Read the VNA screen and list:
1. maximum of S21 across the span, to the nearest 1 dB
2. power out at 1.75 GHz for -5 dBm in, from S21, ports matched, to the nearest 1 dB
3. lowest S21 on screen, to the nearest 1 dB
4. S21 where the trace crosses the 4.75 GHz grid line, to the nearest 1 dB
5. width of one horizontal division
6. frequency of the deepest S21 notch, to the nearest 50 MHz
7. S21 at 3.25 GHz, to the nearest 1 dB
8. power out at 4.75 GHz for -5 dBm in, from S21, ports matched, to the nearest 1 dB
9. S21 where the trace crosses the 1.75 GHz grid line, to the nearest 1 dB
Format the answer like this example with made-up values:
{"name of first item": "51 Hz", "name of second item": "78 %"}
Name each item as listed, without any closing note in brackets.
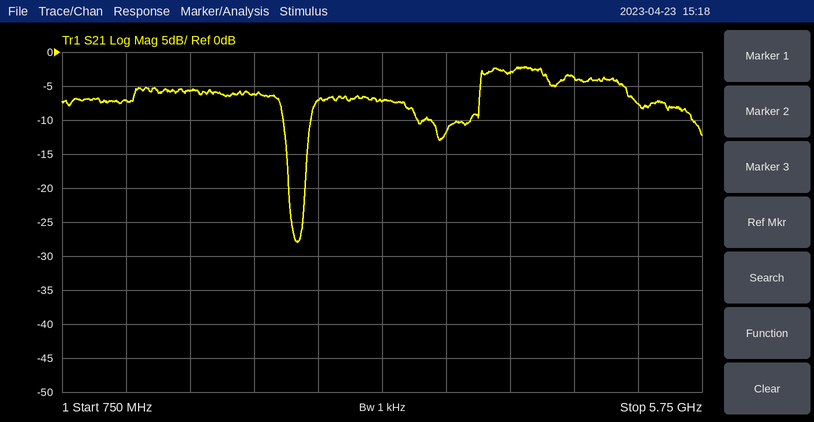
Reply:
{"maximum of S21 across the span, to the nearest 1 dB": "-2 dB", "power out at 1.75 GHz for -5 dBm in, from S21, ports matched, to the nearest 1 dB": "-11 dBm", "lowest S21 on screen, to the nearest 1 dB": "-28 dB", "S21 where the trace crosses the 4.75 GHz grid line, to the nearest 1 dB": "-4 dB", "width of one horizontal division": "500 MHz", "frequency of the deepest S21 notch, to the nearest 50 MHz": "2.60 GHz", "S21 at 3.25 GHz, to the nearest 1 dB": "-7 dB", "power out at 4.75 GHz for -5 dBm in, from S21, ports matched, to the nearest 1 dB": "-9 dBm", "S21 where the trace crosses the 1.75 GHz grid line, to the nearest 1 dB": "-6 dB"}
